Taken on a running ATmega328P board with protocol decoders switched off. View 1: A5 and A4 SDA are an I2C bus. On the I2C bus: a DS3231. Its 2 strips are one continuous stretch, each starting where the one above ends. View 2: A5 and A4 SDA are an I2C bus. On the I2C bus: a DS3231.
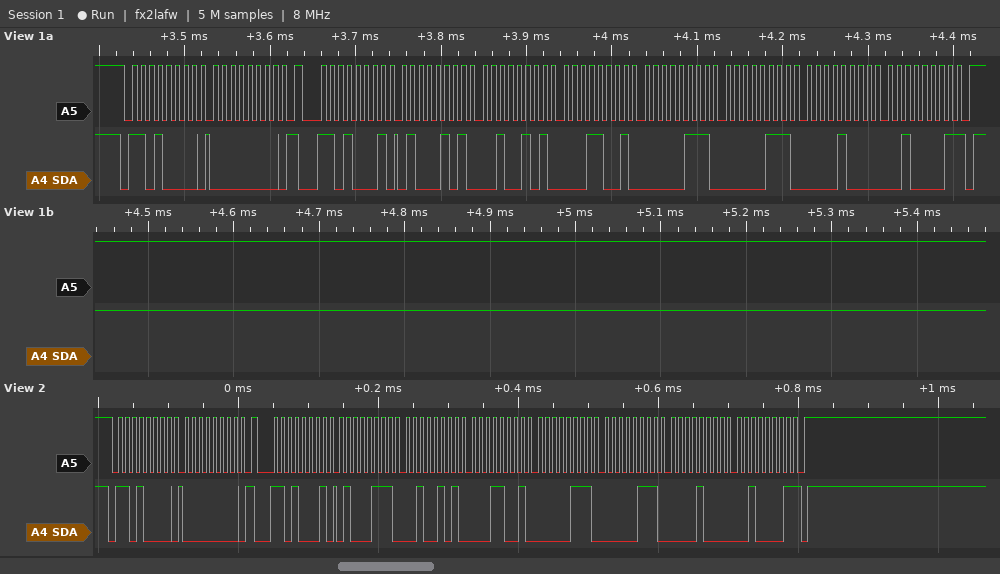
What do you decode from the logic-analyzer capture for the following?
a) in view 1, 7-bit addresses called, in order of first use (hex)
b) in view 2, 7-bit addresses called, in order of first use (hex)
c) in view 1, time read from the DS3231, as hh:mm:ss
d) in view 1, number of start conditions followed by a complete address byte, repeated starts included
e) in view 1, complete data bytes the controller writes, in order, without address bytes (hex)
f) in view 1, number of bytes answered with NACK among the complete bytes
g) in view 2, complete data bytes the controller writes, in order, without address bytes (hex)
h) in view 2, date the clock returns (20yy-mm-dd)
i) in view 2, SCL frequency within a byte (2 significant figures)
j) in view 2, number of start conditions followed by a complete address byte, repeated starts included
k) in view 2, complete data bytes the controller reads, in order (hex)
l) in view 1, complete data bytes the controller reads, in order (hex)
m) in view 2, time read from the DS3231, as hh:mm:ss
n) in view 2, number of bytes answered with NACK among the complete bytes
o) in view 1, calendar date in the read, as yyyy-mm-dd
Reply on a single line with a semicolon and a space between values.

0x68; 0x68; 19:25:45; 2; 00; 1; 00; 2021-08-07; 100 kHz; 2; 47 25 19 07 07 08 21; 45 25 19 07 07 08 21; 19:25:47; 1; 2021-08-07
